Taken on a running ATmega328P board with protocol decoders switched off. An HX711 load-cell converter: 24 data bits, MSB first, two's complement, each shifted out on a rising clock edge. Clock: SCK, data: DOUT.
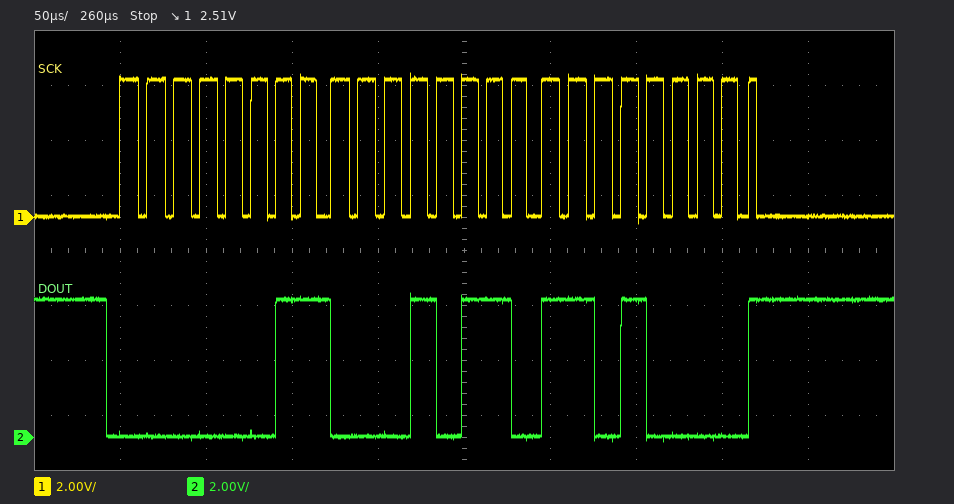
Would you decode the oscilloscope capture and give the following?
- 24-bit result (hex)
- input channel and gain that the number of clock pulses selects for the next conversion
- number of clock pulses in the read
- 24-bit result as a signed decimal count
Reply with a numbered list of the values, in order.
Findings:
1. 0x0316D0
2. channel A, gain 128
3. 25
4. 202448
